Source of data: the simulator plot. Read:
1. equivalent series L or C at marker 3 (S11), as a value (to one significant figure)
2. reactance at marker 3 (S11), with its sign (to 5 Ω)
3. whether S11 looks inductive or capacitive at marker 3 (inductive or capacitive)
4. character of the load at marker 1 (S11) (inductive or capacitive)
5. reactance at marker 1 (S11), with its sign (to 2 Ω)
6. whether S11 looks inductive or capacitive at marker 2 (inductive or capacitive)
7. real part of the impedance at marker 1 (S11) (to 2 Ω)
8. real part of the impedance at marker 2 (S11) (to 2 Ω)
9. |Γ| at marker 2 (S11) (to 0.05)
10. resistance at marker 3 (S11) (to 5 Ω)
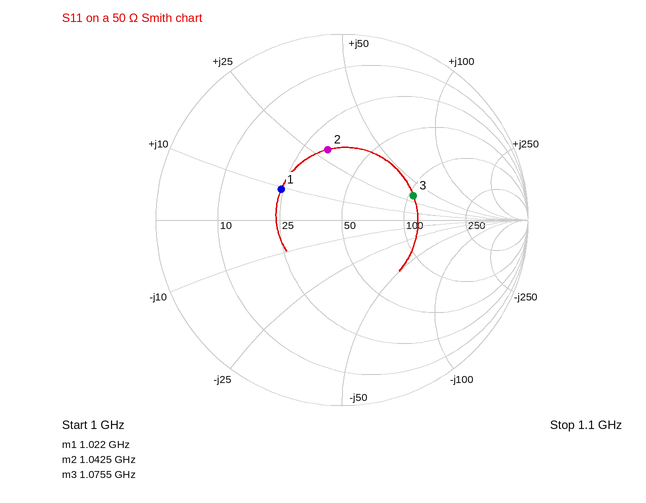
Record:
5 nH
+35 Ω
inductive
inductive
+10 Ω
inductive
24 Ω
32 Ω
0.40
105 Ω
